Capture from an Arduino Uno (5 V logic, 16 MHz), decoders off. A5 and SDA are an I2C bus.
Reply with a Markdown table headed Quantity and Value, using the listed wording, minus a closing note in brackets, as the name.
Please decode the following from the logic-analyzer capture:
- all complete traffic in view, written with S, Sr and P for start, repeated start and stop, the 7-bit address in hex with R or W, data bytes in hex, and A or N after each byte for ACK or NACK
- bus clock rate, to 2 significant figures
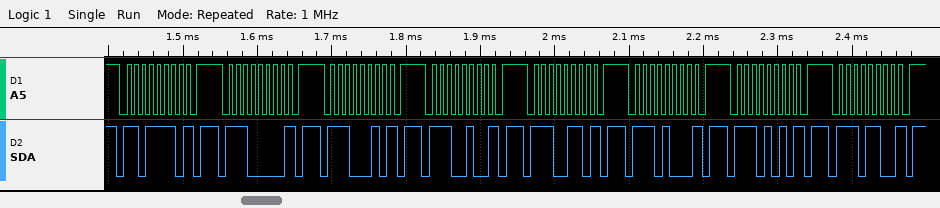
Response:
| Quantity | Value |
|---|---|
| all complete traffic in view, written with S, Sr and P for start, repeated start and stop, the 7-bit address in hex with R or W, data bytes in hex, and A or N after each byte for ACK or NACK | S 6FW N P S 70W N P S 71W N P S 72W N P S 73W N P S 74W N P S 75W N P S 76W N P |
| bus clock rate, to 2 significant figures | 100 kHz |
